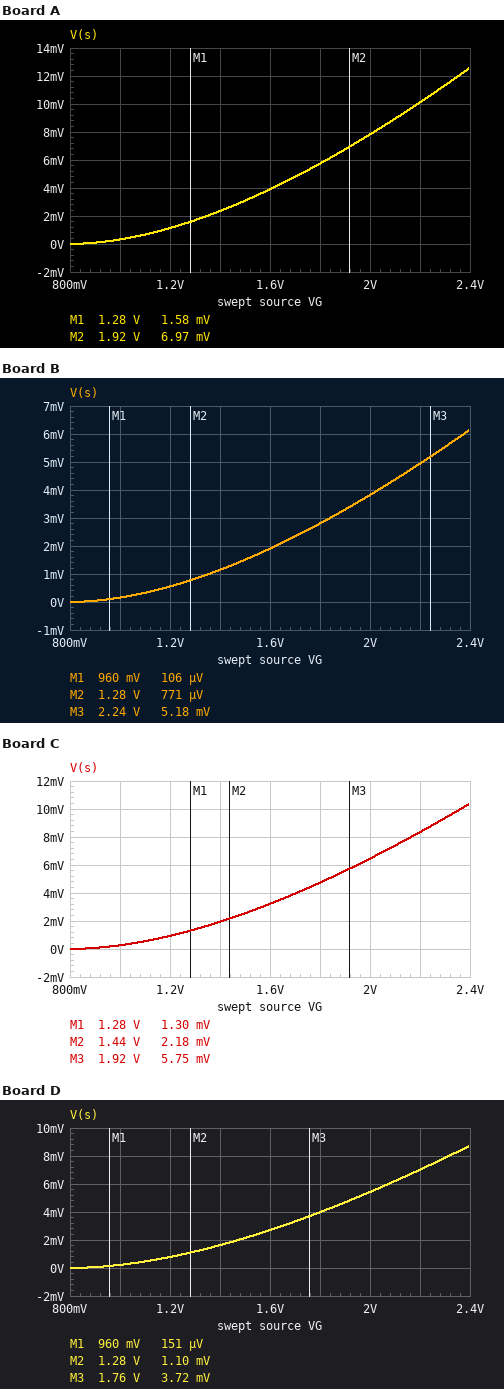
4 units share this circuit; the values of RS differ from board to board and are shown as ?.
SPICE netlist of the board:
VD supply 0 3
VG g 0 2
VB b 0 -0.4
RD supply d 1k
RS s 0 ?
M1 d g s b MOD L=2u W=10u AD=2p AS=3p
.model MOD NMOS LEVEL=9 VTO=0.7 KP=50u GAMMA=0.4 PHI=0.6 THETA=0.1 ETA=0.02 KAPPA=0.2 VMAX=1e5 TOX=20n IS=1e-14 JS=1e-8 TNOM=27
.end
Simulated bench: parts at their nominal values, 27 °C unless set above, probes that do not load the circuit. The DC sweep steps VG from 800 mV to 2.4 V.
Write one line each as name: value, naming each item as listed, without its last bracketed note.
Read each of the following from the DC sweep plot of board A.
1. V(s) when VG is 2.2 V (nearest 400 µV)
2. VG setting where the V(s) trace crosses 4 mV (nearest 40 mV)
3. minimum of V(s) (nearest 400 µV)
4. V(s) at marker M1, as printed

V(s) when VG is 2.2 V: 10.0 mV
VG setting where the V(s) trace crosses 4 mV: 1.60 V
minimum of V(s): 0 V
V(s) at marker M1, as printed: 1.58 mV
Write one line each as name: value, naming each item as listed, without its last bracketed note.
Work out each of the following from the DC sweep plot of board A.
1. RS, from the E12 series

RS, from the E12 series: 68 Ω
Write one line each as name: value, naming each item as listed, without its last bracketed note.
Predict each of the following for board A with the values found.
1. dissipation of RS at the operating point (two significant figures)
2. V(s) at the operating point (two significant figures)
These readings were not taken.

dissipation of RS at the operating point: 900 nW
V(s) at the operating point: 7.8 mV
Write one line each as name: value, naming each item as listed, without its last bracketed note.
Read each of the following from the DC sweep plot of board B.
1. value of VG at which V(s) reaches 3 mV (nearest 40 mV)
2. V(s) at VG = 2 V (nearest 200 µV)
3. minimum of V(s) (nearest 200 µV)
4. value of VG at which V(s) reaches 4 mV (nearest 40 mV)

value of VG at which V(s) reaches 3 mV: 1.84 V
V(s) at VG = 2 V: 3.8 mV
minimum of V(s): 0 V
value of VG at which V(s) reaches 4 mV: 2.04 V
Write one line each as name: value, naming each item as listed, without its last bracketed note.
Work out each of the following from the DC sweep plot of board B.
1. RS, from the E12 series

RS, from the E12 series: 33 Ω
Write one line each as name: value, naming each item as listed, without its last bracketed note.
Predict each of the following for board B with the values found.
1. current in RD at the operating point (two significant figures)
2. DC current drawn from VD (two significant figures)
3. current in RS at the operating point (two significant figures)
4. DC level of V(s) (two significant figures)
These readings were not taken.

current in RD at the operating point: 120 µA
DC current drawn from VD: 120 µA
current in RS at the operating point: 120 µA
DC level of V(s): 3.8 mV
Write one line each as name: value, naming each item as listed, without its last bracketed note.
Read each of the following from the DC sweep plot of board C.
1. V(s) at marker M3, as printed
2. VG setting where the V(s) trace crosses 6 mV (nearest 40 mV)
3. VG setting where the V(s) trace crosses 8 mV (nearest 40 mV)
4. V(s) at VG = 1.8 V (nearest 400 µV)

V(s) at marker M3, as printed: 5.75 mV
VG setting where the V(s) trace crosses 6 mV: 1.96 V
VG setting where the V(s) trace crosses 8 mV: 2.16 V
V(s) at VG = 1.8 V: 4.8 mV
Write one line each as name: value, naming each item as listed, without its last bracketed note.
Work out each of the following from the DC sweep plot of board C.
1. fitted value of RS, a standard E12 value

fitted value of RS, a standard E12 value: 56 Ω
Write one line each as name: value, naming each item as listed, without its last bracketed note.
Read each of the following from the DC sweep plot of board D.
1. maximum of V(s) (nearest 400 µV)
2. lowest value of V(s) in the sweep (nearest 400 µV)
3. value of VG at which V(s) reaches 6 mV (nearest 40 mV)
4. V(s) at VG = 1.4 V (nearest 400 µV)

maximum of V(s): 8.8 mV
lowest value of V(s) in the sweep: 0 V
value of VG at which V(s) reaches 6 mV: 2.08 V
V(s) at VG = 1.4 V: 1.6 mV
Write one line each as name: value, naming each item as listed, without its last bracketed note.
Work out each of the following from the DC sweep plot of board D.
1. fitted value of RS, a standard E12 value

fitted value of RS, a standard E12 value: 47 Ω
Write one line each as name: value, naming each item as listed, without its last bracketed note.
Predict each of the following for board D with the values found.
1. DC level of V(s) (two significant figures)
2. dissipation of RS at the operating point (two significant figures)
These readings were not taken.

DC level of V(s): 5.4 mV
dissipation of RS at the operating point: 630 nW
